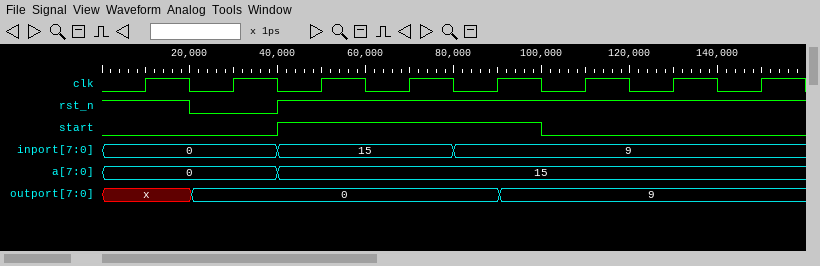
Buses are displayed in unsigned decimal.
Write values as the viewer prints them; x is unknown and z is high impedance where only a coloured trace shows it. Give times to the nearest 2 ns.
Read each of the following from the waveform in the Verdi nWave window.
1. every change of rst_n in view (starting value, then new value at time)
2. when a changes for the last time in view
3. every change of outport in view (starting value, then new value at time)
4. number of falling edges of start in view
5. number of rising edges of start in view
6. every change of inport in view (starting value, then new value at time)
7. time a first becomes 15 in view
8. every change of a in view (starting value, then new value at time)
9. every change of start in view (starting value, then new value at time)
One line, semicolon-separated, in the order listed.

1, 0 at 20 ns, 1 at 40 ns; 40 ns; x, 0 at 20 ns, 9 at 90 ns; 1; 1; 0, 15 at 40 ns, 9 at 80 ns; 40 ns; 0, 15 at 40 ns; 0, 1 at 40 ns, 0 at 100 ns
